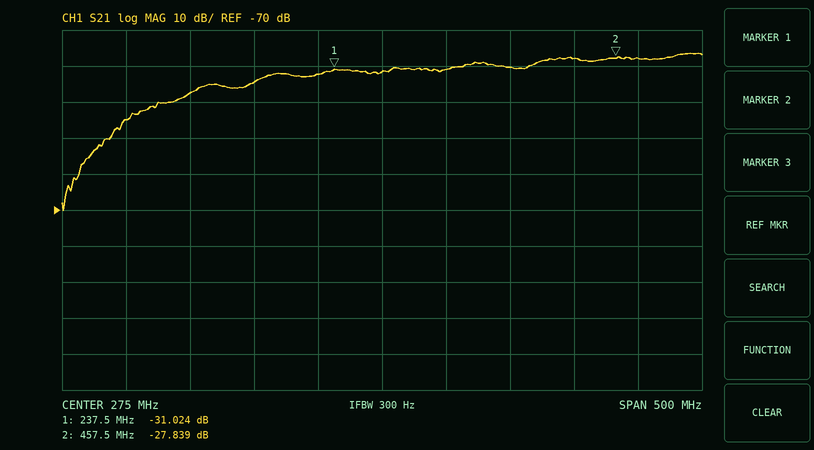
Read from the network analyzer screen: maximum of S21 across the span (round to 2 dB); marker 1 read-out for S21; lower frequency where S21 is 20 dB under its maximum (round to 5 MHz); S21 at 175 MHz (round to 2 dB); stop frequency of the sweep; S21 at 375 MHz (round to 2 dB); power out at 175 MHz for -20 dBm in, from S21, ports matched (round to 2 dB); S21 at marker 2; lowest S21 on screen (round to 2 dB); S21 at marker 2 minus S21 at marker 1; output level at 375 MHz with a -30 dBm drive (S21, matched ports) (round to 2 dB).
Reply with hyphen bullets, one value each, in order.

- -26 dB
- -31.024 dB
- 70 MHz
- -34 dB
- 525 MHz
- -30 dB
- -54 dBm
- -27.839 dB
- -70 dB
- 3.185 dB
- -60 dBm
